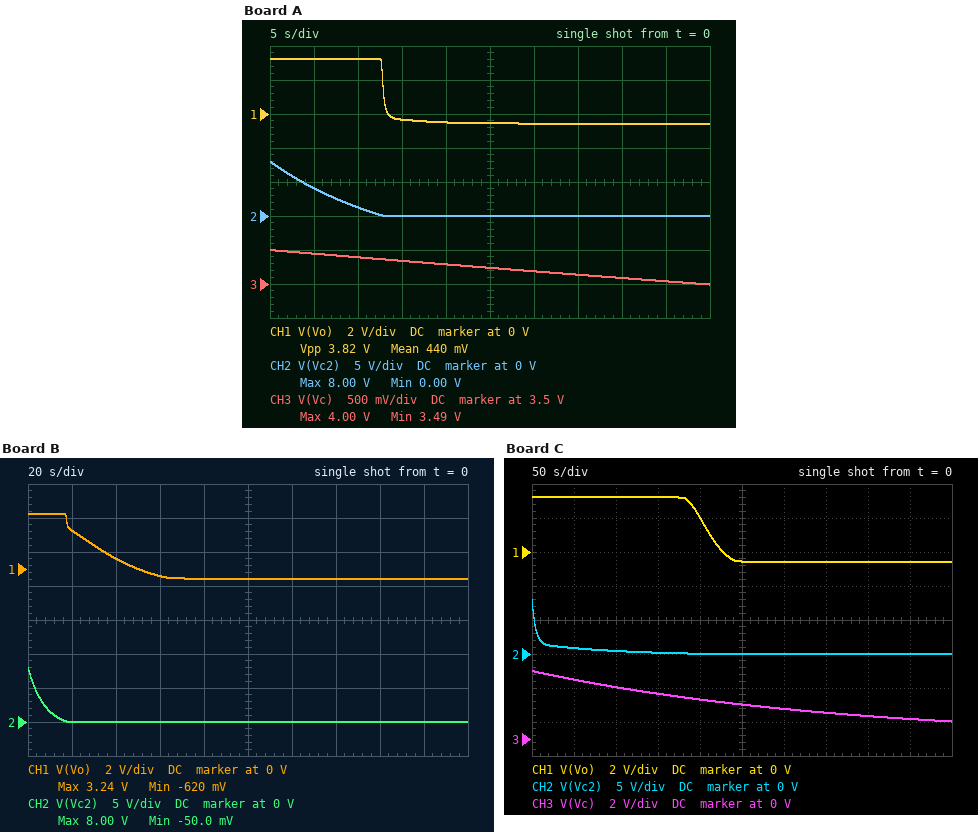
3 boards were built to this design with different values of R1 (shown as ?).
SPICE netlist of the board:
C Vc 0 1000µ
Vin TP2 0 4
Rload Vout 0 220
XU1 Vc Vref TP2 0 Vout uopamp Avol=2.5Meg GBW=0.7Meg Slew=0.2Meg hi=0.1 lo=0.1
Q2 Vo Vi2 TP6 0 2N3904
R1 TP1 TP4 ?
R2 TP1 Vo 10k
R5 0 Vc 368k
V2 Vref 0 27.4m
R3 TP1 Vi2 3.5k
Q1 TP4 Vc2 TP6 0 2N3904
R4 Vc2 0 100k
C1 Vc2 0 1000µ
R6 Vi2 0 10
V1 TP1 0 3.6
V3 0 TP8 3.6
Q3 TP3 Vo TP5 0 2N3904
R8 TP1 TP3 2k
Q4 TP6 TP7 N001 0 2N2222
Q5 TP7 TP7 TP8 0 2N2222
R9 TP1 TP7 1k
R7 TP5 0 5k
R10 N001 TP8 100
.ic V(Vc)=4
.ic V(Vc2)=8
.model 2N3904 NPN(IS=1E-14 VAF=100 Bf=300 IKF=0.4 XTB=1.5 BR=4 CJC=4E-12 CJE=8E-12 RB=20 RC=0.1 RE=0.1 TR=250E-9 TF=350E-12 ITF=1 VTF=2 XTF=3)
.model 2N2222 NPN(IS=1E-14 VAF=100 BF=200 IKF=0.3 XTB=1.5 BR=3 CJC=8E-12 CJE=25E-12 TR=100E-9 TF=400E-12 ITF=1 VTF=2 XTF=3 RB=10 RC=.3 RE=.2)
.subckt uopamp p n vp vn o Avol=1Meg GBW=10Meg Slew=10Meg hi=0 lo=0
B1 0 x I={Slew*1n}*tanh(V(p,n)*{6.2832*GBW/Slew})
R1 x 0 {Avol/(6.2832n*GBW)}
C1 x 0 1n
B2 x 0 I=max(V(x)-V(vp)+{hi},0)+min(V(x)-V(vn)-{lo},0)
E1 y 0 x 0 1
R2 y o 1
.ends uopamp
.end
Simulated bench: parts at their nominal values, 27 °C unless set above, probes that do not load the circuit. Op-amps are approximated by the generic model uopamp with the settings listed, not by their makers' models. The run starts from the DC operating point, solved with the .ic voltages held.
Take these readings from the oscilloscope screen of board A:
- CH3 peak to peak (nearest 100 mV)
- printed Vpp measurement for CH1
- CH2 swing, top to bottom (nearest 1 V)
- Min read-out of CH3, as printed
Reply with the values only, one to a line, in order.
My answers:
500 mV
3.82 V
8 V
3.49 V
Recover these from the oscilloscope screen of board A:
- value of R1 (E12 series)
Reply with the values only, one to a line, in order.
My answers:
18 kΩ
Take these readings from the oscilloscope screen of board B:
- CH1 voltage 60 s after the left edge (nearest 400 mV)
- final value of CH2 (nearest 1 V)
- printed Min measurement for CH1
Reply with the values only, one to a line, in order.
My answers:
-400 mV
0 V
-620 mV
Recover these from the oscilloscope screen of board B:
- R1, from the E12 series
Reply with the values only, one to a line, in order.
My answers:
8.2 kΩ
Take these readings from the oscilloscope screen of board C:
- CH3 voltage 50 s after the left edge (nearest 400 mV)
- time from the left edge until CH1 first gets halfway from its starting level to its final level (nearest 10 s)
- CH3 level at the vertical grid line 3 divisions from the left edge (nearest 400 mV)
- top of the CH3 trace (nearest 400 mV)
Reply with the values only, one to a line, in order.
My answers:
3.6 V
210 s
2.8 V
4.0 V
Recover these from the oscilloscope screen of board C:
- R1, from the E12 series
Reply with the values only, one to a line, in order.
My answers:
4.7 kΩ
